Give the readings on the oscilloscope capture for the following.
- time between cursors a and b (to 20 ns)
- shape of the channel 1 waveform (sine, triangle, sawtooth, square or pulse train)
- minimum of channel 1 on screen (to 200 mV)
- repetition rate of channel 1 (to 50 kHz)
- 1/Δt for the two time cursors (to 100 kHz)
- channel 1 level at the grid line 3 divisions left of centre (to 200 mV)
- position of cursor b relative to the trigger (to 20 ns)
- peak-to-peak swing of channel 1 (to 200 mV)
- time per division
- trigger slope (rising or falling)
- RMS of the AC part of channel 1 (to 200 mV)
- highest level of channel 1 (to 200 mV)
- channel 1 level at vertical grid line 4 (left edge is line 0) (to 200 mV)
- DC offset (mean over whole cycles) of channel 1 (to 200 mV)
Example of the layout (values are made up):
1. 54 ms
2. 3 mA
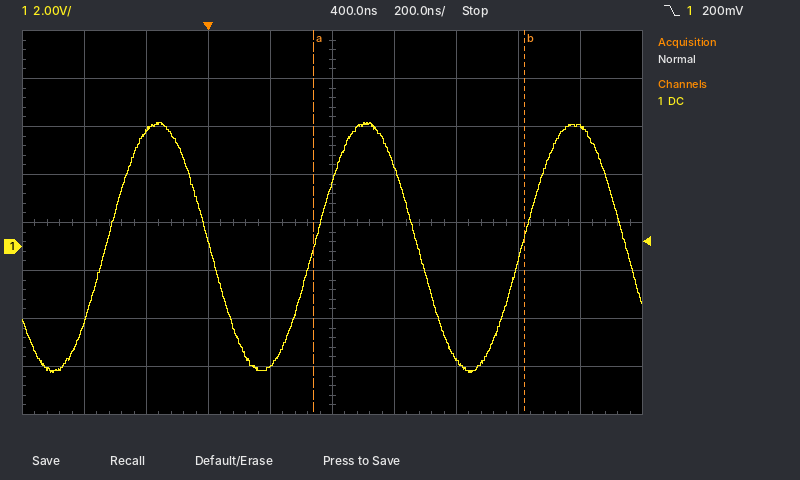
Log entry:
1. 680 ns
2. sine
3. -5.2 V
4. 1.50 MHz
5. 1.5 MHz
6. 4.8 V
7. +1.02 µs
8. 10.4 V
9. 200 ns
10. falling
11. 3.6 V
12. 5.2 V
13. -5.0 V
14. 0.0 V
